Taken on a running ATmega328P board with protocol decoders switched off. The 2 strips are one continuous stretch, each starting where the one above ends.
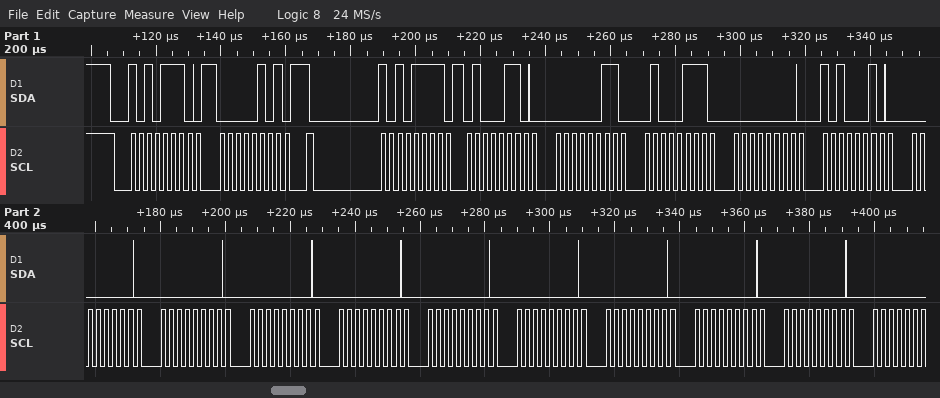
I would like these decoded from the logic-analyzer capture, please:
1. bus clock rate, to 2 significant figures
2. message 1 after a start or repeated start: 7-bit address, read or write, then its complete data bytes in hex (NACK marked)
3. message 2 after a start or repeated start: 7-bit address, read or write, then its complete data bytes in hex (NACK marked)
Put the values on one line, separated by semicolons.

400 kHz; 0x57 write: 05; 0x57 read: 46 03 47 00 A2 00 00 00 00 00 00 00 00 00
